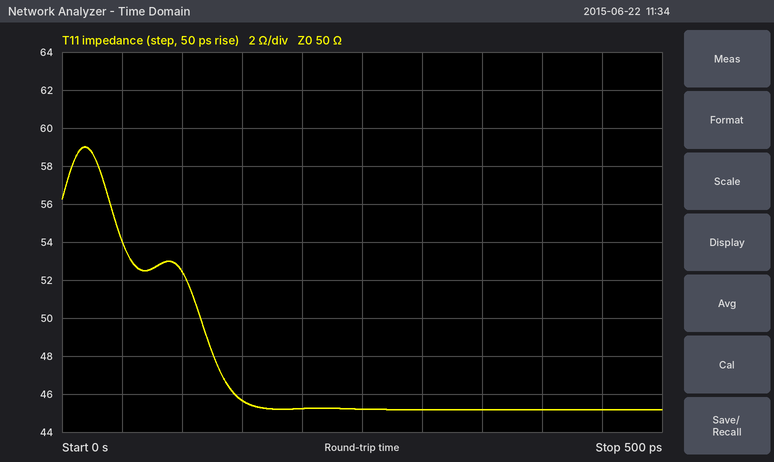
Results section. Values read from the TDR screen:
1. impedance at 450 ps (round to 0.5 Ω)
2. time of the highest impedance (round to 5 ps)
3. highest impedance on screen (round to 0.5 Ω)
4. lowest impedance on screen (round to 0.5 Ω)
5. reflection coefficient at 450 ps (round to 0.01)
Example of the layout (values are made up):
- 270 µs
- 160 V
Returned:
- 45.0 Ω
- 20 ps
- 59.0 Ω
- 45.0 Ω
- -0.05
